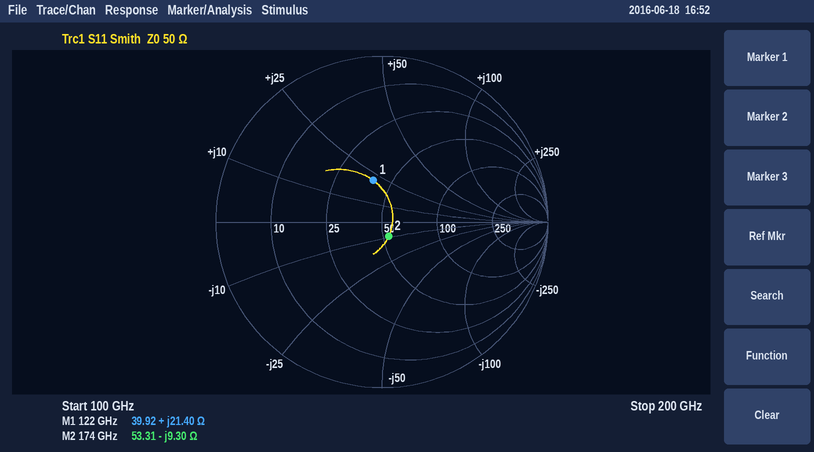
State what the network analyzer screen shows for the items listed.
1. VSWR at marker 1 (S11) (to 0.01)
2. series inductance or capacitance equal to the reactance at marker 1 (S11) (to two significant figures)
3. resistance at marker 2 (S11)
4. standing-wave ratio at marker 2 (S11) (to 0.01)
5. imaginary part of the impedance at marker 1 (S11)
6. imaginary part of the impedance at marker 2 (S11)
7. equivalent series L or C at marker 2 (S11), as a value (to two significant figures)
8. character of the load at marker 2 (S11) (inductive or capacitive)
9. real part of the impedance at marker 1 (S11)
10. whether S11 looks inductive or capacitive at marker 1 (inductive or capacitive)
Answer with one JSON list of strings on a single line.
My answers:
["1.69", "28 pH", "53.31 Ω", "1.21", "+21.40 Ω", "-9.30 Ω", "98 fF", "capacitive", "39.92 Ω", "inductive"]
